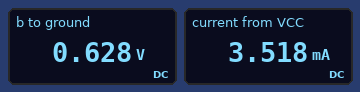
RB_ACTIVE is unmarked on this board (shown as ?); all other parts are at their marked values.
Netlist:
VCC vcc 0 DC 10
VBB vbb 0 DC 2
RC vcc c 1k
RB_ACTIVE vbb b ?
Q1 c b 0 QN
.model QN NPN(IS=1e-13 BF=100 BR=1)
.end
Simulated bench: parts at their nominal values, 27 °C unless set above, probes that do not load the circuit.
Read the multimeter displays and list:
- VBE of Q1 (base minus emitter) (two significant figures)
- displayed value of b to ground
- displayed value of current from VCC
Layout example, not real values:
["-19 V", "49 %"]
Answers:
["630 mV", "0.628 V", "3.518 mA"]
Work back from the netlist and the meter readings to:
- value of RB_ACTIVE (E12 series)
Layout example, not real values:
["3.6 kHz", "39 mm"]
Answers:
["39 kΩ"]
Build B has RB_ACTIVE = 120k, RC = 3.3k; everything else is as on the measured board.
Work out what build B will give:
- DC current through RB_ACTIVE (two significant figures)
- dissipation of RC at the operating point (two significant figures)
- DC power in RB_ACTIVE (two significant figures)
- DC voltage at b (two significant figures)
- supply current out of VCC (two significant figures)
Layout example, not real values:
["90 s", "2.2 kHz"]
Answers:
["12 µA", "4.5 mW", "16 µW", "600 mV", "1.2 mA"]
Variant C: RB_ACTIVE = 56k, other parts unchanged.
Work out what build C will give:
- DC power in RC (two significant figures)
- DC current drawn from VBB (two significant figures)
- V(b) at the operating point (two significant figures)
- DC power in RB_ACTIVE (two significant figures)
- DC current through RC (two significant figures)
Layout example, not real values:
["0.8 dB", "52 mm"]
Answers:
["6.1 mW", "25 µA", "620 mV", "34 µW", "2.5 mA"]
